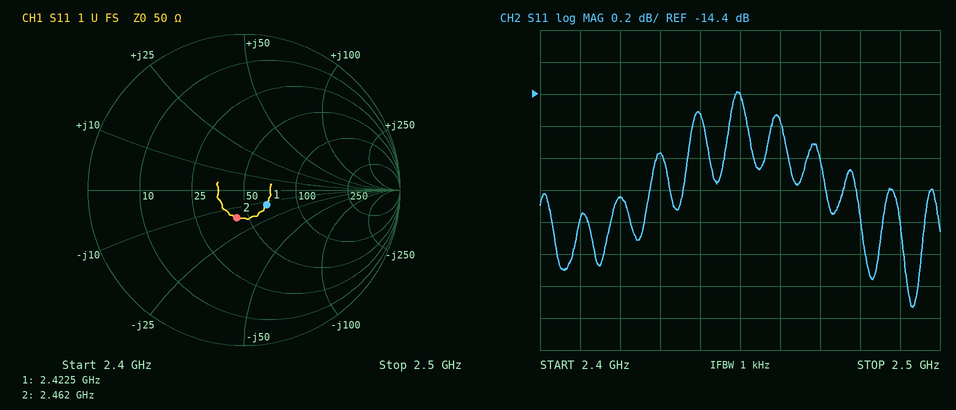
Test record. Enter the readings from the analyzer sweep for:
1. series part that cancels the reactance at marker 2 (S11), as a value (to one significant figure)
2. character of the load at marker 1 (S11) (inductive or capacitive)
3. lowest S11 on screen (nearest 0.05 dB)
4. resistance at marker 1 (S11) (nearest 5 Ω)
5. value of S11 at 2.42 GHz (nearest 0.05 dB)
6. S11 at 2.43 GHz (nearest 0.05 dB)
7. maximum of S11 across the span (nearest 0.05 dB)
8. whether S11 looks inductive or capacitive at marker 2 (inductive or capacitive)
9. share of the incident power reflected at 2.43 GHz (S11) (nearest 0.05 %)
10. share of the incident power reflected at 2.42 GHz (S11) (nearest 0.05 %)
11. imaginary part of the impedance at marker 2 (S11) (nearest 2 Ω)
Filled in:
1 nH
capacitive
-15.75 dB
65 Ω
-15.05 dB
-14.75 dB
-14.40 dB
capacitive
3.35 %
3.15 %
-16 Ω
